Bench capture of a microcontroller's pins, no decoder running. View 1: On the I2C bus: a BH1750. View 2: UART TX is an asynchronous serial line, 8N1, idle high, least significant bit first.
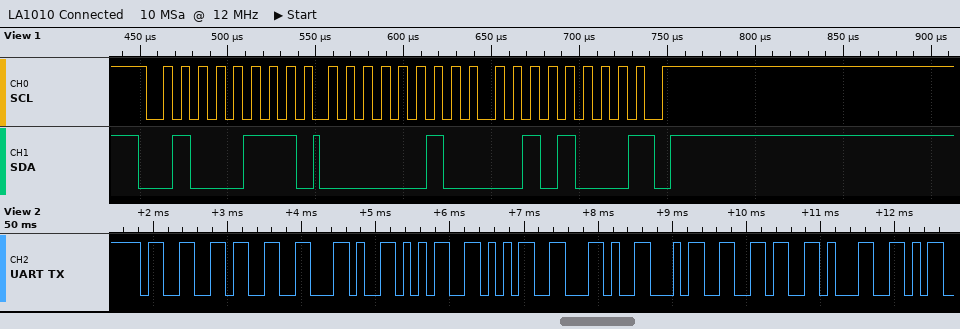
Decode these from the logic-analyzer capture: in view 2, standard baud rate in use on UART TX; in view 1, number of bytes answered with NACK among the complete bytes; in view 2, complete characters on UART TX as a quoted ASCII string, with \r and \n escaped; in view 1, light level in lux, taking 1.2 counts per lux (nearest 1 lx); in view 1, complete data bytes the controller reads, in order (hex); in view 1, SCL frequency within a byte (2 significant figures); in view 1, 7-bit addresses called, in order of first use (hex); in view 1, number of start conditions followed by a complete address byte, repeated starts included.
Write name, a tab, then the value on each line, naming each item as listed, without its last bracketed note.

in view 2, standard baud rate in use on UART TX	9600 baud
in view 1, number of bytes answered with NACK among the complete bytes	1
in view 2, complete characters on UART TX as a quoted ASCII string, with \r and \n escaped	"33,55,461"
in view 1, light level in lux, taking 1.2 counts per lux	460 lx
in view 1, complete data bytes the controller reads, in order	02 28
in view 1, SCL frequency within a byte	100 kHz
in view 1, 7-bit addresses called, in order of first use	0x23
in view 1, number of start conditions followed by a complete address byte, repeated starts included	1
